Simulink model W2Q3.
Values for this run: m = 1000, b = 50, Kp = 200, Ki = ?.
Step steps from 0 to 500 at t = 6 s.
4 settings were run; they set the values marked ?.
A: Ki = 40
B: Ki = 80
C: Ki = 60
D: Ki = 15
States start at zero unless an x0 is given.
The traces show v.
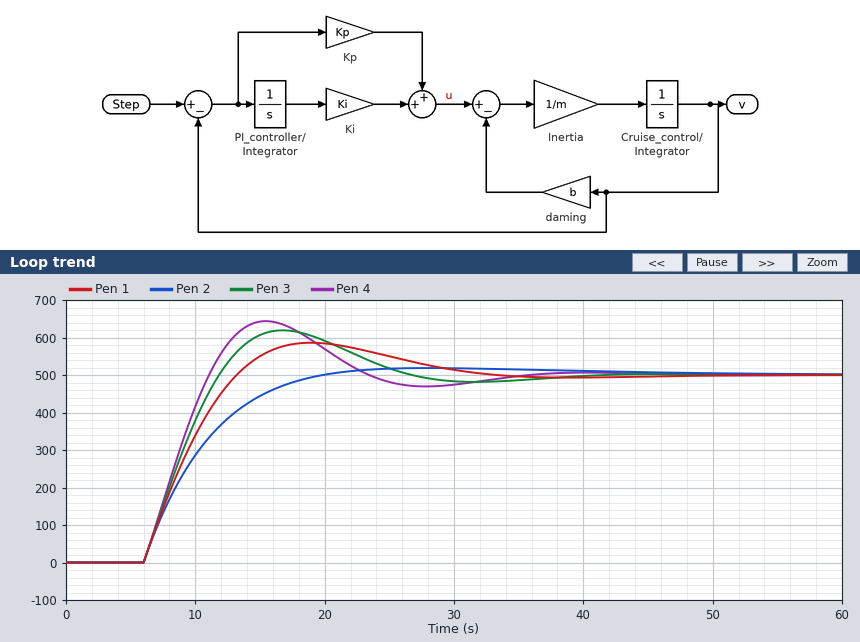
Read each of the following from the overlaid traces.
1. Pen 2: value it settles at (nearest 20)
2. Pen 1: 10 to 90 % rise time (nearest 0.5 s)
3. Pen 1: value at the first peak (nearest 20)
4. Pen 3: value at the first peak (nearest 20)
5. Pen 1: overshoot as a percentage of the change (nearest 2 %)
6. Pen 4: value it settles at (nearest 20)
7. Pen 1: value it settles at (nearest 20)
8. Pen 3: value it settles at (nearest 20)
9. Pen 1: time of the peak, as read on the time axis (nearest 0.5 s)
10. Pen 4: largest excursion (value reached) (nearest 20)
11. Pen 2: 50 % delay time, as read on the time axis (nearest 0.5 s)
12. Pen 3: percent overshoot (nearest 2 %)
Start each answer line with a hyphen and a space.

- 500
- 5.5 s
- 580
- 620
- 18 %
- 500
- 500
- 500
- 19.0 s
- 640
- 9.5 s
- 24 %
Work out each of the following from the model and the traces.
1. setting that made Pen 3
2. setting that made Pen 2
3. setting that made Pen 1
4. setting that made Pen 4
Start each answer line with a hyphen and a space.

- C
- D
- A
- B
